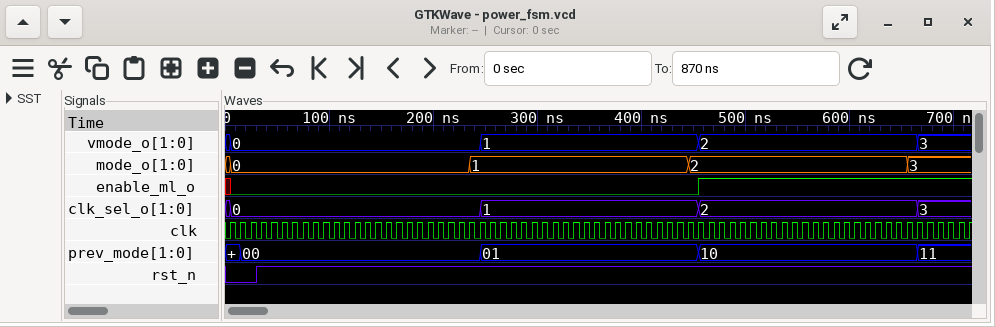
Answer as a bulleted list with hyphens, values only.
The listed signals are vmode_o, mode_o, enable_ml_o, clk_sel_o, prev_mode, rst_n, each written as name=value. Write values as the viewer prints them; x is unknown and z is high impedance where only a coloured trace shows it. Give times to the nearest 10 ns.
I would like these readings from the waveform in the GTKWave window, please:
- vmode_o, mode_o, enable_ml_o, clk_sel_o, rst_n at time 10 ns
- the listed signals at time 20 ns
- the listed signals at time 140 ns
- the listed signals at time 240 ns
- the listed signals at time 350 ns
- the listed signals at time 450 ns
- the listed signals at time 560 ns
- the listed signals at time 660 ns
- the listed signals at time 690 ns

- vmode_o=0, mode_o=0, enable_ml_o=0, clk_sel_o=0, rst_n=0
- vmode_o=0, mode_o=0, enable_ml_o=0, clk_sel_o=0, prev_mode=00, rst_n=0
- vmode_o=0, mode_o=0, enable_ml_o=0, clk_sel_o=0, prev_mode=00, rst_n=1
- vmode_o=0, mode_o=1, enable_ml_o=0, clk_sel_o=0, prev_mode=00, rst_n=1
- vmode_o=1, mode_o=1, enable_ml_o=0, clk_sel_o=1, prev_mode=01, rst_n=1
- vmode_o=1, mode_o=2, enable_ml_o=0, clk_sel_o=1, prev_mode=01, rst_n=1
- vmode_o=2, mode_o=2, enable_ml_o=1, clk_sel_o=2, prev_mode=10, rst_n=1
- vmode_o=2, mode_o=3, enable_ml_o=1, clk_sel_o=2, prev_mode=10, rst_n=1
- vmode_o=3, mode_o=3, enable_ml_o=1, clk_sel_o=3, prev_mode=11, rst_n=1
